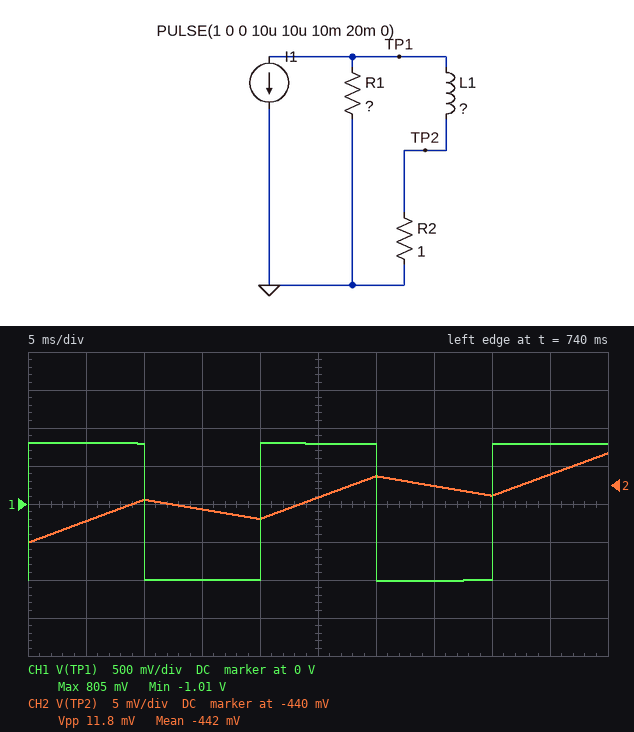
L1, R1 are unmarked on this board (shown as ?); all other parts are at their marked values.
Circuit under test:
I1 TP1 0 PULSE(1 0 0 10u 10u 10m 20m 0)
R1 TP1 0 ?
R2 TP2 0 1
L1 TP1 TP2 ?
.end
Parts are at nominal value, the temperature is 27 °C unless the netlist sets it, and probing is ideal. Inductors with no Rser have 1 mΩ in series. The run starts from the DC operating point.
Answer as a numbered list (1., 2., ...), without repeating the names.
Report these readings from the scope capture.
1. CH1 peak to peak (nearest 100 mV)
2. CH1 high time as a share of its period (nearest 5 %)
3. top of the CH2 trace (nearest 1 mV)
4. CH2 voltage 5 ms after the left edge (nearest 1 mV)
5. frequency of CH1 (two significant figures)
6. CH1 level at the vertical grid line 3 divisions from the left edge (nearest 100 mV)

1. 1.8 V
2. 50 %
3. -436 mV
4. -445 mV
5. 50 Hz
6. -1.0 V
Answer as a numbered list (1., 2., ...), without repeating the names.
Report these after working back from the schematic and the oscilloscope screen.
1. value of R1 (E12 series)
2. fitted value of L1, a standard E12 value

1. 1.8 Ω
2. 2.2 H
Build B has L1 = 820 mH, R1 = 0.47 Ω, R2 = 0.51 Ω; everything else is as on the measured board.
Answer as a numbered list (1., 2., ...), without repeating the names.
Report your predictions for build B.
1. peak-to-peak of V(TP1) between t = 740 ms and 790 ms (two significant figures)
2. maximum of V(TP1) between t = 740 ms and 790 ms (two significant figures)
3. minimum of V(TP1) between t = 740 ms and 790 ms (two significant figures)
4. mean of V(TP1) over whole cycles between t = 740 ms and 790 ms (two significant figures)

1. 470 mV
2. 160 mV
3. -310 mV
4. -77 mV
